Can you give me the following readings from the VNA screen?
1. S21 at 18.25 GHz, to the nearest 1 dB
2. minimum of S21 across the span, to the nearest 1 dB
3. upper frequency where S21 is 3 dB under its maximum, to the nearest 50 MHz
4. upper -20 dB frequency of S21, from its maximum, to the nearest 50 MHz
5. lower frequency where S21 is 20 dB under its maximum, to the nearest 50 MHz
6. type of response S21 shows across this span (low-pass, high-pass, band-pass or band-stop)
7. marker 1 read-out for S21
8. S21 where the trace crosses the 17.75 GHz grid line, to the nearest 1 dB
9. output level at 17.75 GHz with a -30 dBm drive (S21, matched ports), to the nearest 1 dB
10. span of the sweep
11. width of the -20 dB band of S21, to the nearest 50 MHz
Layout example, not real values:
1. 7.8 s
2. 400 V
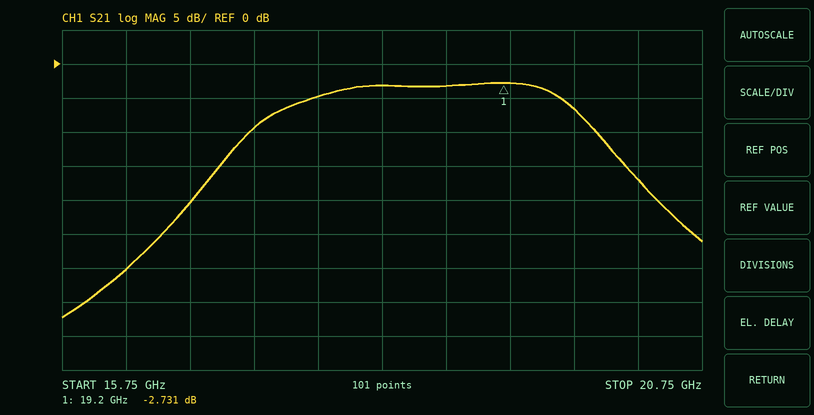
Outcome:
1. -3 dB
2. -37 dB
3. 19.70 GHz
4. 20.55 GHz
5. 16.65 GHz
6. band-pass
7. -2.731 dB
8. -5 dB
9. -35 dBm
10. 5 GHz
11. 3.90 GHz
